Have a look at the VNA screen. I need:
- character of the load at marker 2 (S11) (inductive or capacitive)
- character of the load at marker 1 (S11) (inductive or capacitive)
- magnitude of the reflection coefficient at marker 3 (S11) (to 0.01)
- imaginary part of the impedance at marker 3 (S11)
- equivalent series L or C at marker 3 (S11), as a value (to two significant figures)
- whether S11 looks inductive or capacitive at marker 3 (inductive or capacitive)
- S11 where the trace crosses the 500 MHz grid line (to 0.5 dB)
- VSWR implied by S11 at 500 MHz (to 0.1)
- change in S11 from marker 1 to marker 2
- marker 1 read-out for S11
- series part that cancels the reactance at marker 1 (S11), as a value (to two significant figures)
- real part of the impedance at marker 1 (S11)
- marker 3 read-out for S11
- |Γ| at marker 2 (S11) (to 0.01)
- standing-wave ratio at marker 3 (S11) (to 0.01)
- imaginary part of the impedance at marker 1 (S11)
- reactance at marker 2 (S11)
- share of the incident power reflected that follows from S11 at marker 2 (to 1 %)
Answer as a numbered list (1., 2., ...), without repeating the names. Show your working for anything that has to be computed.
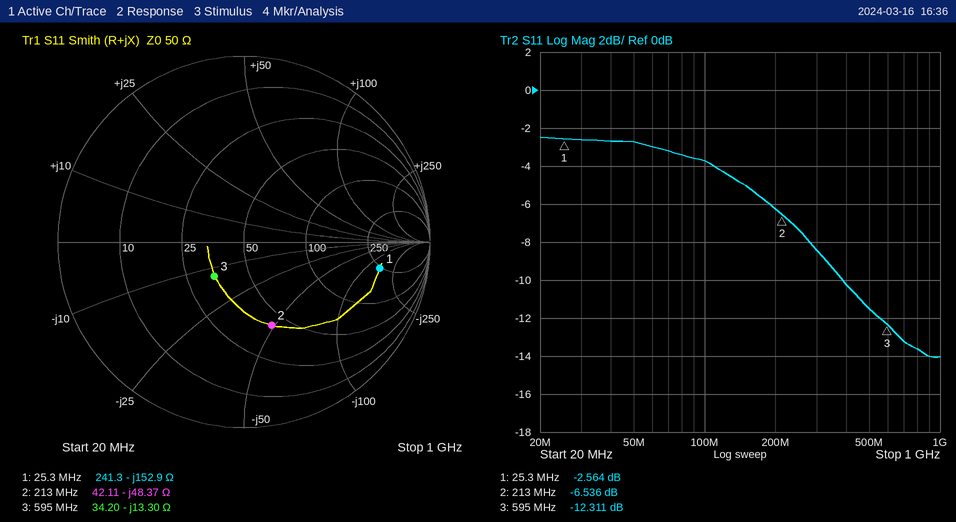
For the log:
1. capacitive
2. capacitive
3. 10^(-12.311/20) ≈ 0.24
4. -13.30 Ω
5. C = 1/(2π × 595 MHz × 13.3 Ω) ≈ 20 pF
6. capacitive
7. -11.5 dB
8. |Γ| = 10^(-11.5/20) = 0.2661; VSWR = (1 + 0.2661)/(1 − 0.2661) ≈ 1.7
9. -6.536 − (-2.564) = -3.972 dB
10. -2.564 dB
11. L = 152.9 Ω/(2π × 25.3 MHz) ≈ 962 nH, so 960 nH to two significant figures
12. 241.3 Ω
13. -12.311 dB
14. 0.47
15. 1.64
16. -152.9 Ω
17. -48.37 Ω
18. 10^(-6.536/10) ≈ 22 %
